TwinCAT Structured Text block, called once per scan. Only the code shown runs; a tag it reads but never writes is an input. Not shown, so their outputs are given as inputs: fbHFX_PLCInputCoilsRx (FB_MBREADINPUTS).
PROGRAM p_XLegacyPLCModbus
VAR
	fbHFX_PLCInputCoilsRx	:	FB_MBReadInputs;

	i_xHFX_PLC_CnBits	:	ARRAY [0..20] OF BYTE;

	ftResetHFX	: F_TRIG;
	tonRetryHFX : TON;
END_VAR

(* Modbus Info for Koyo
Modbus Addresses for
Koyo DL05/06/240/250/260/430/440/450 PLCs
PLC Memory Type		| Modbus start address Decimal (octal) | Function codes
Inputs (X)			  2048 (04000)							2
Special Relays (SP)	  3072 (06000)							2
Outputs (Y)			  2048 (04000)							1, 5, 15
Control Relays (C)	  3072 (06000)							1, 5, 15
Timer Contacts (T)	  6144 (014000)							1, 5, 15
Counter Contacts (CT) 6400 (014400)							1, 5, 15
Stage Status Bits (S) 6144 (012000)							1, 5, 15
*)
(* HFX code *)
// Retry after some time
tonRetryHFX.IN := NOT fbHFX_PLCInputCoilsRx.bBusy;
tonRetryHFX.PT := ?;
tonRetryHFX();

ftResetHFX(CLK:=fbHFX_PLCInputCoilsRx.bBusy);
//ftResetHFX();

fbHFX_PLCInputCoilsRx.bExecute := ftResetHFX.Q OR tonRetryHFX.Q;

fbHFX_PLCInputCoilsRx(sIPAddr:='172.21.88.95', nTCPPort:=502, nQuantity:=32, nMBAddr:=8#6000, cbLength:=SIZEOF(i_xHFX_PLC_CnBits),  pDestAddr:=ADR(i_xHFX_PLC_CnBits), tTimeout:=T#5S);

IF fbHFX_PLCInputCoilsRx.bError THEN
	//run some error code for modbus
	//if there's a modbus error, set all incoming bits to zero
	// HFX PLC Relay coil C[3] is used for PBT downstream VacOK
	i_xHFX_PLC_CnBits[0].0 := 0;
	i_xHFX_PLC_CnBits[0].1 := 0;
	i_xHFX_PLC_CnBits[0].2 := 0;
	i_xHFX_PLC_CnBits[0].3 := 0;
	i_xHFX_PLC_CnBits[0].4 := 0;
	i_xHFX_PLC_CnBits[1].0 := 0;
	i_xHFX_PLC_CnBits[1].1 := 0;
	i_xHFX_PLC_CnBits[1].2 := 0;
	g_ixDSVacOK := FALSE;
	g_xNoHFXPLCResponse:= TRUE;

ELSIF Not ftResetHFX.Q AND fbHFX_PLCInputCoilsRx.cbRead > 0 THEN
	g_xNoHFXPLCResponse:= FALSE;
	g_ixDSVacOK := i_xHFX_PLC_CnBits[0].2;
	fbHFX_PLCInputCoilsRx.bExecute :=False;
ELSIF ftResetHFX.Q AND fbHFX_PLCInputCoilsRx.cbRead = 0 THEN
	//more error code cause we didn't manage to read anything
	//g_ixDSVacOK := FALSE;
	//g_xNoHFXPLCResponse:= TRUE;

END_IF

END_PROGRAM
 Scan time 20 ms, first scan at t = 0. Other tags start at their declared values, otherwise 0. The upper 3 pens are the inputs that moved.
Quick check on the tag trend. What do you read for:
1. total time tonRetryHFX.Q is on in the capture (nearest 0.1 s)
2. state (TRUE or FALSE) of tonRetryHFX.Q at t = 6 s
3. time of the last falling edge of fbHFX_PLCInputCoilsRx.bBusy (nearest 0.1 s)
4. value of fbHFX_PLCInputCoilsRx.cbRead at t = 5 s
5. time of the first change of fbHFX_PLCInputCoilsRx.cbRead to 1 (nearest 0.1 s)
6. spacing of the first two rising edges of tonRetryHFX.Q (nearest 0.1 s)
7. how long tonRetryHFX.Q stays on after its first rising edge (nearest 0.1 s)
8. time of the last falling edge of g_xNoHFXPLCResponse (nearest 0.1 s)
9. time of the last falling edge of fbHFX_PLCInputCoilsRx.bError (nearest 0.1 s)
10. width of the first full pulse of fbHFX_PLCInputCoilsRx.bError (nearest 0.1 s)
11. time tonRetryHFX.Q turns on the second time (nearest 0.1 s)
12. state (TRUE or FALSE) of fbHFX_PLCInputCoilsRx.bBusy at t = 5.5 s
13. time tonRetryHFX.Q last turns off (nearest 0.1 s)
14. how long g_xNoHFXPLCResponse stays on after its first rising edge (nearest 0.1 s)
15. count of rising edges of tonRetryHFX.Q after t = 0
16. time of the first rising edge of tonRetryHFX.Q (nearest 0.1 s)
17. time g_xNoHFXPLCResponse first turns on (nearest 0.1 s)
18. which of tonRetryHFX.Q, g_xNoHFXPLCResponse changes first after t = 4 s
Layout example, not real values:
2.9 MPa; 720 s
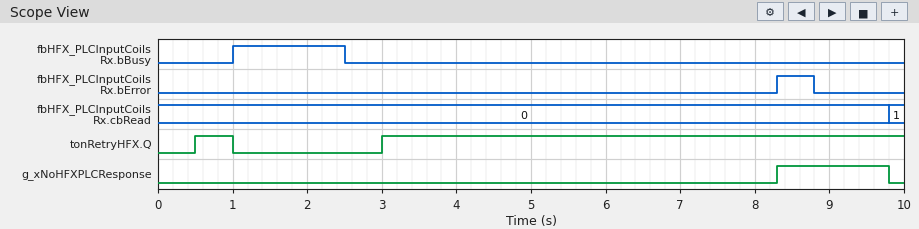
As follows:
7.5 s; TRUE; 2.5 s; 0; 9.8 s; 2.5 s; 0.5 s; 9.8 s; 8.8 s; 0.5 s; 3.0 s; FALSE; 1.0 s; 1.5 s; 2; 0.5 s; 8.3 s; g_xNoHFXPLCResponse
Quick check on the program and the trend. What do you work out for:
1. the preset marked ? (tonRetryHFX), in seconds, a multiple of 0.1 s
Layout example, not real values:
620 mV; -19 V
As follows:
0.5 s
